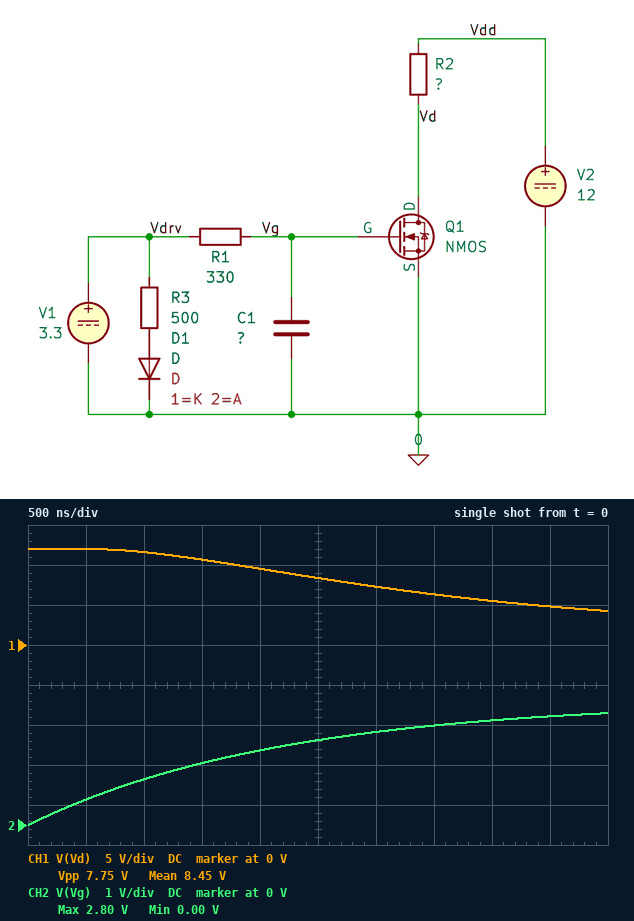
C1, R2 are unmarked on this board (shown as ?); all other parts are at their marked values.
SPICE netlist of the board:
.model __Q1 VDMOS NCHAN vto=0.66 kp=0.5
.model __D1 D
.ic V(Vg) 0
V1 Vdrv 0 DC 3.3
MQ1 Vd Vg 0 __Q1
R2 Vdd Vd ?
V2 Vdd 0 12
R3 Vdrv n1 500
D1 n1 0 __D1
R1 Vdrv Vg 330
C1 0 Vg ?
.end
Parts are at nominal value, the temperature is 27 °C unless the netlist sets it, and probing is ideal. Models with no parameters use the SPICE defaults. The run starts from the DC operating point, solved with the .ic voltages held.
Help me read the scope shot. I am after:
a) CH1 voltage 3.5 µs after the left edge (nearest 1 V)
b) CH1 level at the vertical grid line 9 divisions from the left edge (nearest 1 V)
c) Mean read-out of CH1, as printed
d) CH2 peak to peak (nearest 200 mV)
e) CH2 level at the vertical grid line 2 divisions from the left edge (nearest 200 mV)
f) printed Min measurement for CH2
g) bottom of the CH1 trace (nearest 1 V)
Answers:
6 V
5 V
8.45 V
2.8 V
1.2 V
0.00 V
4 V
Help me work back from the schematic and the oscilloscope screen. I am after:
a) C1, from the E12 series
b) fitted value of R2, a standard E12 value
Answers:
5.6 nF
6.8 Ω
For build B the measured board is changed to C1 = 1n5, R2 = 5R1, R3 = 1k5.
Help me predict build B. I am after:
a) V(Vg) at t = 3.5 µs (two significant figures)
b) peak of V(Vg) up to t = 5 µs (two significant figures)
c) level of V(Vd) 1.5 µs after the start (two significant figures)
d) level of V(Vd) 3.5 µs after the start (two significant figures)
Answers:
3.1 V
3.2 V
7.8 V
4.6 V
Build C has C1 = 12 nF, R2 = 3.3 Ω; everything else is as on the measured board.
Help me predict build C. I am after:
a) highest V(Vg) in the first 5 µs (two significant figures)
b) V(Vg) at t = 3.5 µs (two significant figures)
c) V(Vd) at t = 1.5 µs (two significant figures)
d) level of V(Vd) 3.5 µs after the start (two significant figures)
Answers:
2.2 V
1.8 V
12 V
11 V
